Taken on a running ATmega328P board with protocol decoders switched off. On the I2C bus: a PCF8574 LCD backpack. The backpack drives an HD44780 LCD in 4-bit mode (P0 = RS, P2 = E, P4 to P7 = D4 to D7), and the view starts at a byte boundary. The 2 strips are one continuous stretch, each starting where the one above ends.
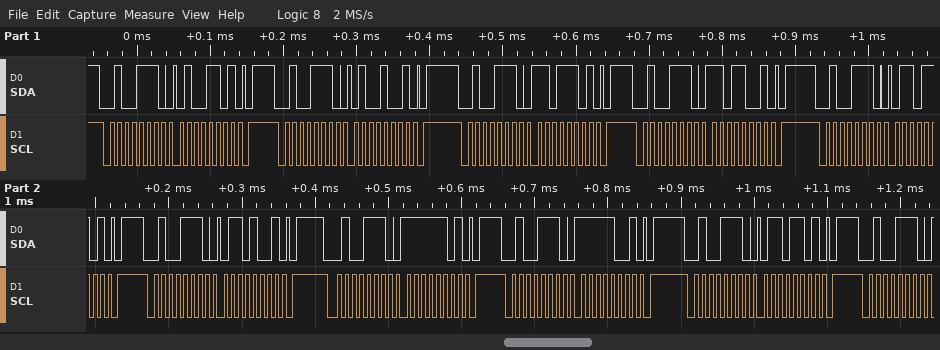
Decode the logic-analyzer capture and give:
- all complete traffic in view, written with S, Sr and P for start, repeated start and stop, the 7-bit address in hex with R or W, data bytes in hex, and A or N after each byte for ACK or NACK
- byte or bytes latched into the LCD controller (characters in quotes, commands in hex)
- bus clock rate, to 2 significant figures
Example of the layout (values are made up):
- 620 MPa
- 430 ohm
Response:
- S 27W A 4D A P S 27W A 49 A P S 27W A DD A P S 27W A D9 A P S 27W A 6D A P S 27W A 69 A P S 27W A FD A P S 27W A F9 A P S 27W A 6D A P S 27W A
- 'M' 'o'
- 100 kHz
